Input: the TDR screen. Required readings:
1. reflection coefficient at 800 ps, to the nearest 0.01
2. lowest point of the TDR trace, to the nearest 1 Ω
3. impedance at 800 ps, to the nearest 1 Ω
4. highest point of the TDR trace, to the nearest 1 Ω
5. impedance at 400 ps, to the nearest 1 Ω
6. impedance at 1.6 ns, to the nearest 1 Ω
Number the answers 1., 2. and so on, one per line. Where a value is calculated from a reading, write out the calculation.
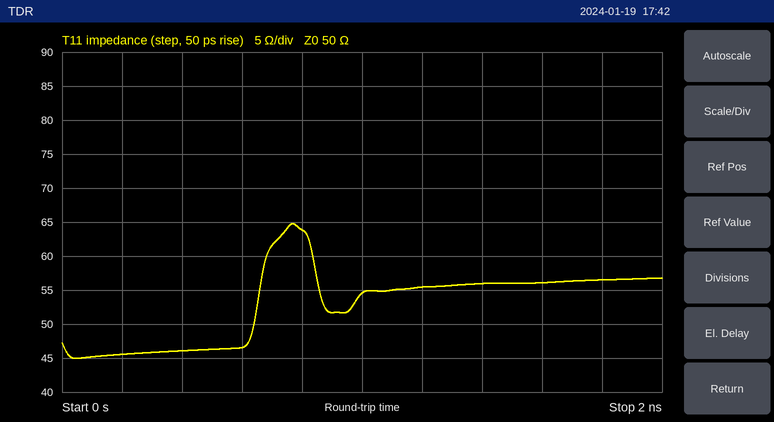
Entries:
1. (64 − 50)/(64 + 50) ≈ +0.12
2. 45 Ω
3. 64 Ω
4. 65 Ω
5. 46 Ω
6. 56 Ω
